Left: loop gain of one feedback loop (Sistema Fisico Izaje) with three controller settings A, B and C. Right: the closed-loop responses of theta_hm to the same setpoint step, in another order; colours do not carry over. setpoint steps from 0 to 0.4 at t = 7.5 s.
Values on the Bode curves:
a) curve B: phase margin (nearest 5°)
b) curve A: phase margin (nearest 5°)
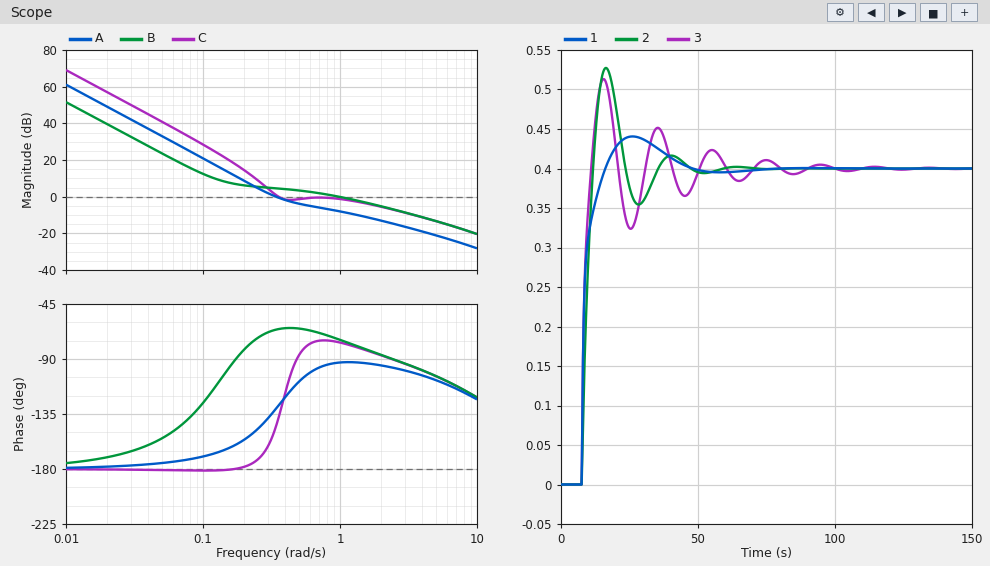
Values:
105°
50°
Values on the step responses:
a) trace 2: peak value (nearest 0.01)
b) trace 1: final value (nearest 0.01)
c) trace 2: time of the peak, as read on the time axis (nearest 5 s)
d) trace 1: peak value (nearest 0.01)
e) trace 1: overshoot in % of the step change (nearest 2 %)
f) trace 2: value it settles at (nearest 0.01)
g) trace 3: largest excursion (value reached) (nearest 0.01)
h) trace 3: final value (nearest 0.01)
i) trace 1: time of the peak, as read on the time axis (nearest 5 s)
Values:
0.53
0.40
15 s
0.44
10 %
0.40
0.51
0.40
25 s
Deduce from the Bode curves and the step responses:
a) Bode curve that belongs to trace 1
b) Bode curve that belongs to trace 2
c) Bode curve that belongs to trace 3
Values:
B
A
C
